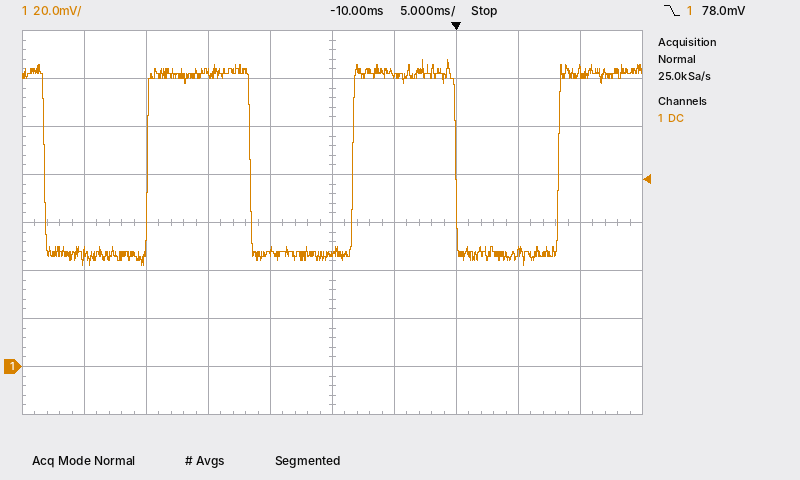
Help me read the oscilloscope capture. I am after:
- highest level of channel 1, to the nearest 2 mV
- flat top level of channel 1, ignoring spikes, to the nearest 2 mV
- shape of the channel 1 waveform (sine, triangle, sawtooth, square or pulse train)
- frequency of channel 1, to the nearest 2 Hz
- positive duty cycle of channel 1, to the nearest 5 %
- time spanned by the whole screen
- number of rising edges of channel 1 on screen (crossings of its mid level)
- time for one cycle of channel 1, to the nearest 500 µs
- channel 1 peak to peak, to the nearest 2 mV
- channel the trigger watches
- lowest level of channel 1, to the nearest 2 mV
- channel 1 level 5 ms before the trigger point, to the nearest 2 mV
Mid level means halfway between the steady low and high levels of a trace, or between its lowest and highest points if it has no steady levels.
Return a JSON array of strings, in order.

["128 mV", "122 mV", "square", "60 Hz", "50 %", "50 ms", "3", "16.5 ms", "86 mV", "channel 1", "42 mV", "122 mV"]
